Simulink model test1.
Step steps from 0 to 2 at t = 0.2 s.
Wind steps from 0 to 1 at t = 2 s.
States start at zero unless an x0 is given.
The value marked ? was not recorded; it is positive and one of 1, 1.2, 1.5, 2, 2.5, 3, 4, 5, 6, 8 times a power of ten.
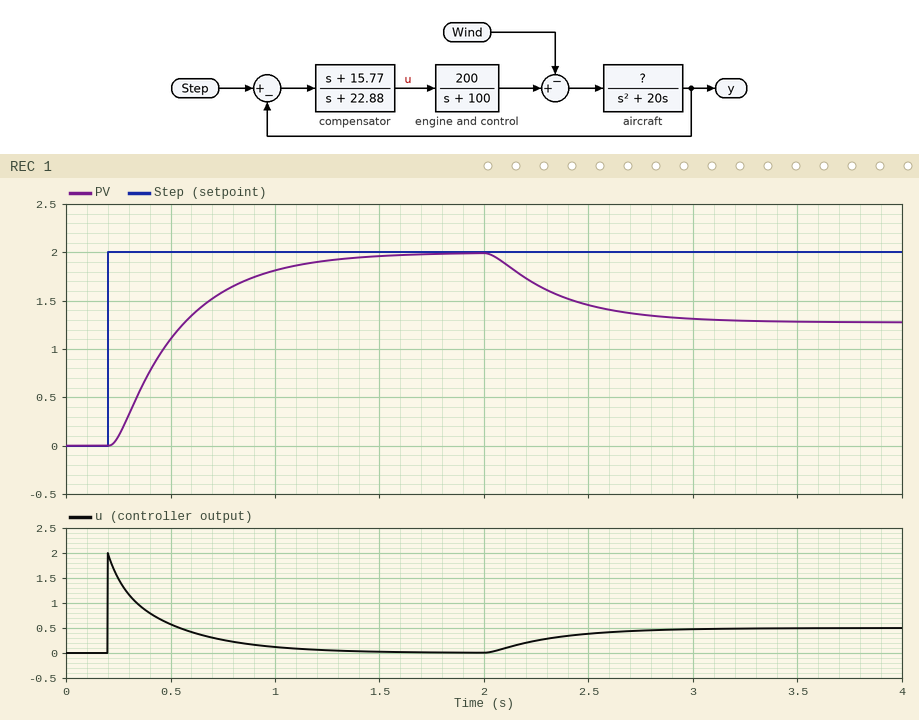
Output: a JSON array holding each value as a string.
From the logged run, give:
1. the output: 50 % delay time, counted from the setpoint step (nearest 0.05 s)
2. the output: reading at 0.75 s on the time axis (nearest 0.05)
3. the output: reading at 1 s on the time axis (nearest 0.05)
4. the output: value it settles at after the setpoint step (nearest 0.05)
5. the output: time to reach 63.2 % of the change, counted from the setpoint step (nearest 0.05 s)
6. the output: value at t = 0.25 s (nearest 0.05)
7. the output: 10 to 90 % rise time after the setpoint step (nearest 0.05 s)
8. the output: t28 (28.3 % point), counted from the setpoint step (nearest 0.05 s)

["0.25 s", "1.60", "1.80", "2.00", "0.35 s", "0.10", "0.70 s", "0.15 s"]
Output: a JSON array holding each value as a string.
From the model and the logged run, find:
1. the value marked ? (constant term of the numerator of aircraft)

["40"]
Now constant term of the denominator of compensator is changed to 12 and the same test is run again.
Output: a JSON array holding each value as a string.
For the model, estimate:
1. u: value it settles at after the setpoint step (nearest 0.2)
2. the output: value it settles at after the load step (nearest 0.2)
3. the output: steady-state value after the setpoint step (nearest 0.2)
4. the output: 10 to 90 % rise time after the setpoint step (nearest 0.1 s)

["0.0", "1.6", "2.0", "0.3 s"]
